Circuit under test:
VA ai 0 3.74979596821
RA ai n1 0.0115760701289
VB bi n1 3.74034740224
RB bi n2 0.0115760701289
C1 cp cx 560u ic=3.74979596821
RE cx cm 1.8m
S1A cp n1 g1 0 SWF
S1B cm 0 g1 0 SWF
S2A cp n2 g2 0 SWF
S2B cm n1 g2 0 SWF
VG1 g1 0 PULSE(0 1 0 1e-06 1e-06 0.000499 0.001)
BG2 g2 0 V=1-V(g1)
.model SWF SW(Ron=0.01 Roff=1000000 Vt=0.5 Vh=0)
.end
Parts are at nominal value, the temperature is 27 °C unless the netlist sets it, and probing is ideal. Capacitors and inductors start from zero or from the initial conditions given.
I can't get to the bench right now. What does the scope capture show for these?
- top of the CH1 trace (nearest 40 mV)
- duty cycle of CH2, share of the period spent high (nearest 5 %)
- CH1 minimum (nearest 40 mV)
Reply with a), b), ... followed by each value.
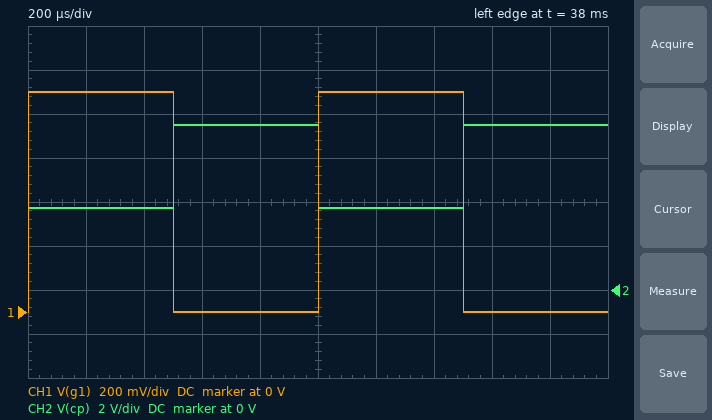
a) 1.00 V
b) 50 %
c) 0 V
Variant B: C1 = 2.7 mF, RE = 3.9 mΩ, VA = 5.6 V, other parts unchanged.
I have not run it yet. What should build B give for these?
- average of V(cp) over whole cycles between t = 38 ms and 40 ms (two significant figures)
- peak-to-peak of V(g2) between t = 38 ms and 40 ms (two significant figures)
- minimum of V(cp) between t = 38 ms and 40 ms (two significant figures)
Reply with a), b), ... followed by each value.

a) 7.5 V
b) 1.0 V
c) 4.5 V
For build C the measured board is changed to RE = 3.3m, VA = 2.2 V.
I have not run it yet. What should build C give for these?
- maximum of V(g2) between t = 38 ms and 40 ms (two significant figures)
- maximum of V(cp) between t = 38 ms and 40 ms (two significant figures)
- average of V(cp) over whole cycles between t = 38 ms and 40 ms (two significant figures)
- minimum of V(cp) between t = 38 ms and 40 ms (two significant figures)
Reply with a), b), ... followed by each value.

a) 1.0 V
b) 5.9 V
c) 4.1 V
d) 2.2 V
